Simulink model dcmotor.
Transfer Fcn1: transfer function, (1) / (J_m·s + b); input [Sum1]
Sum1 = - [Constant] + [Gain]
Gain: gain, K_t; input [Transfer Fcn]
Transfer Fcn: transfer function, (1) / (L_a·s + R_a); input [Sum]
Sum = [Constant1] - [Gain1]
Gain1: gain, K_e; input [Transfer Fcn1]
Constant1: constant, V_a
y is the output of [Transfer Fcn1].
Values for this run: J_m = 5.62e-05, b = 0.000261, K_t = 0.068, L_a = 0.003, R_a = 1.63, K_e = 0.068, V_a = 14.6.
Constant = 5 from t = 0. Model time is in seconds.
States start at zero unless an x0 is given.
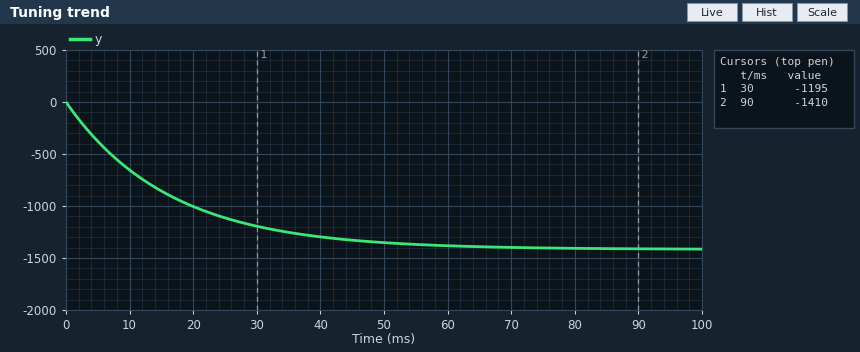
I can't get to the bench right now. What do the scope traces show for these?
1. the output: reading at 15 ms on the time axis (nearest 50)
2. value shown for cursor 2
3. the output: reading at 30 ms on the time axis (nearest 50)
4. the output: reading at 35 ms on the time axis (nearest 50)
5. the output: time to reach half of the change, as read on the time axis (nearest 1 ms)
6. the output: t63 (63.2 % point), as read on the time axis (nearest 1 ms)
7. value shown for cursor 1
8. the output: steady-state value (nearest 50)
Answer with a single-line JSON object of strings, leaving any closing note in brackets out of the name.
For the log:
{"the output: reading at 15 ms on the time axis": "-850", "value shown for cursor 2": "-1410", "the output: reading at 30 ms on the time axis": "-1200", "the output: reading at 35 ms on the time axis": "-1250", "the output: time to reach half of the change, as read on the time axis": "11 ms", "the output: t63 (63.2 % point), as read on the time axis": "16 ms", "value shown for cursor 1": "-1195", "the output: steady-state value": "-1400"}
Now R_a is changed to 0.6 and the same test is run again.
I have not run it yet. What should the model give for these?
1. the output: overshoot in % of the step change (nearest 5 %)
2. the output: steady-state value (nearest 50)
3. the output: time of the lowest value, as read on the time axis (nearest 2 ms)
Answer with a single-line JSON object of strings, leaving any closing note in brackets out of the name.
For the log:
{"the output: overshoot in % of the step change": "25 %", "the output: steady-state value": "-400", "the output: time of the lowest value, as read on the time axis": "14 ms"}
